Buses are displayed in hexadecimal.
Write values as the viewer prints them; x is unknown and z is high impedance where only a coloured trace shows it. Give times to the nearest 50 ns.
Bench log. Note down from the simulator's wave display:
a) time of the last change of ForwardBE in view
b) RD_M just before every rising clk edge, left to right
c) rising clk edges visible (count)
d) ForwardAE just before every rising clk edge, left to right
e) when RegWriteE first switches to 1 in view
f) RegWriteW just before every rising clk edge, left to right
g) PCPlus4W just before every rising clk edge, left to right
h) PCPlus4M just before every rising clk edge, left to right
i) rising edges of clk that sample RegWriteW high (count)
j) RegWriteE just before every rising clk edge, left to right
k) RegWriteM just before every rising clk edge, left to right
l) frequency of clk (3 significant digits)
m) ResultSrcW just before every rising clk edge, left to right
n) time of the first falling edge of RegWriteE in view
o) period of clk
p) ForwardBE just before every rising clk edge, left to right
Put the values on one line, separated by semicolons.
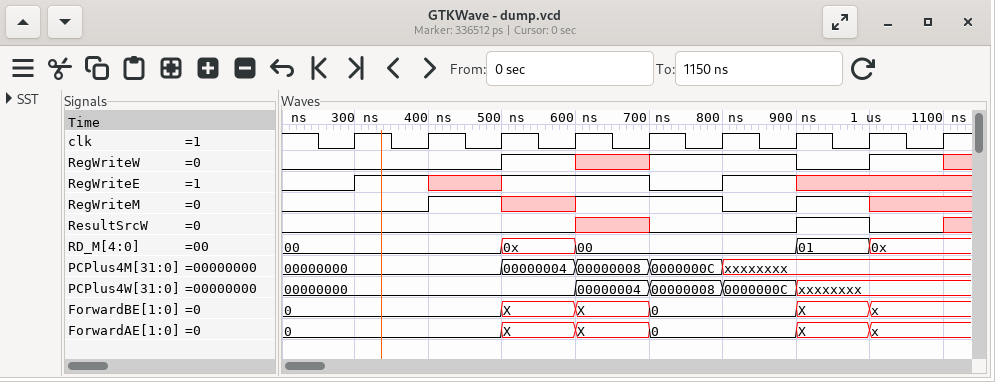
1000 ns; 00, 00, 00, 0x, 00, 00, 00, 01, 0x; 9; 0, 0, 0, X, X, 0, 0, X, x; 300 ns; 0 0 0 1 x 1 1 0 1; 00000000, 00000000, 00000000, 00000000, 00000004, 00000008, 0000000C, xxxxxxxx, xxxxxxxx; 00000000, 00000000, 00000000, 00000004, 00000008, 0000000C, xxxxxxxx, xxxxxxxx, xxxxxxxx; 4; 0 1 x 1 1 0 1 x x; 0 0 1 x 1 1 0 1 x; 10.0 MHz; 0 0 0 0 x 0 0 1 0; 700 ns; 100 ns; 0, 0, 0, X, X, 0, 0, X, x
